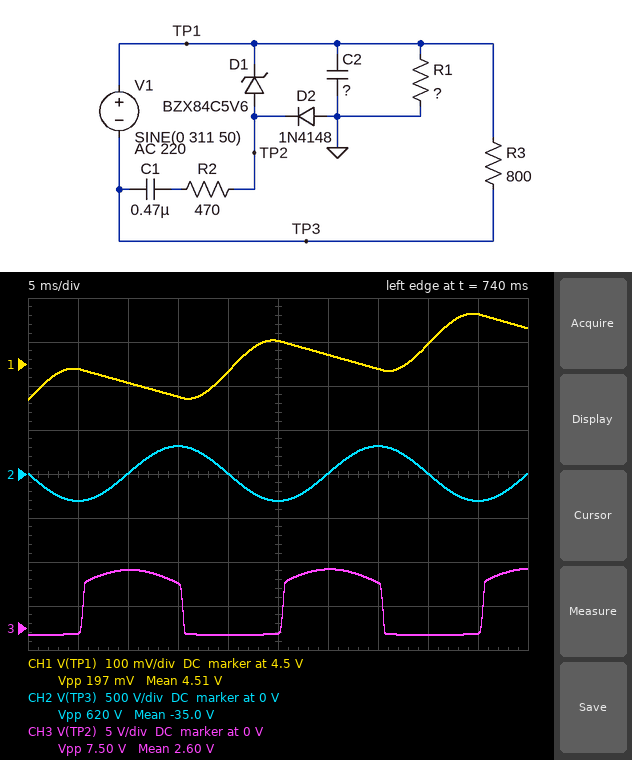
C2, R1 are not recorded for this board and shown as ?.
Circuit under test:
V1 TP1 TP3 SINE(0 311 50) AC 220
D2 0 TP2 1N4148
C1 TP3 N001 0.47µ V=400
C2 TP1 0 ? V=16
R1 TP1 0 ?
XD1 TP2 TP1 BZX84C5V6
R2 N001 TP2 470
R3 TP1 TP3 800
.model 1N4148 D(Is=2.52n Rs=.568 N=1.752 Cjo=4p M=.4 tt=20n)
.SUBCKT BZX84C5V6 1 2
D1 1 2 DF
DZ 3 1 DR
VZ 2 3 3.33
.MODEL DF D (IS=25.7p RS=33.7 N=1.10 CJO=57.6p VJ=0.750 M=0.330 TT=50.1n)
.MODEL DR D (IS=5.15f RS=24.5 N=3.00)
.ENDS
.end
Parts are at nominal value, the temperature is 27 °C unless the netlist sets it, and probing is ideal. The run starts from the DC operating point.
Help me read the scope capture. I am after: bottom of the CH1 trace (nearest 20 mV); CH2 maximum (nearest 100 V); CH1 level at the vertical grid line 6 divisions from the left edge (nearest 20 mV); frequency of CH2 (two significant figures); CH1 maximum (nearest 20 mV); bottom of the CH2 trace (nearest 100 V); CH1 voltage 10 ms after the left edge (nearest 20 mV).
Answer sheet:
4.42 V
300 V
4.52 V
50 Hz
4.62 V
-300 V
4.46 V
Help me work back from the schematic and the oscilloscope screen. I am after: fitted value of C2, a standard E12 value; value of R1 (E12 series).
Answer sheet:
1.5 mF
470 Ω
